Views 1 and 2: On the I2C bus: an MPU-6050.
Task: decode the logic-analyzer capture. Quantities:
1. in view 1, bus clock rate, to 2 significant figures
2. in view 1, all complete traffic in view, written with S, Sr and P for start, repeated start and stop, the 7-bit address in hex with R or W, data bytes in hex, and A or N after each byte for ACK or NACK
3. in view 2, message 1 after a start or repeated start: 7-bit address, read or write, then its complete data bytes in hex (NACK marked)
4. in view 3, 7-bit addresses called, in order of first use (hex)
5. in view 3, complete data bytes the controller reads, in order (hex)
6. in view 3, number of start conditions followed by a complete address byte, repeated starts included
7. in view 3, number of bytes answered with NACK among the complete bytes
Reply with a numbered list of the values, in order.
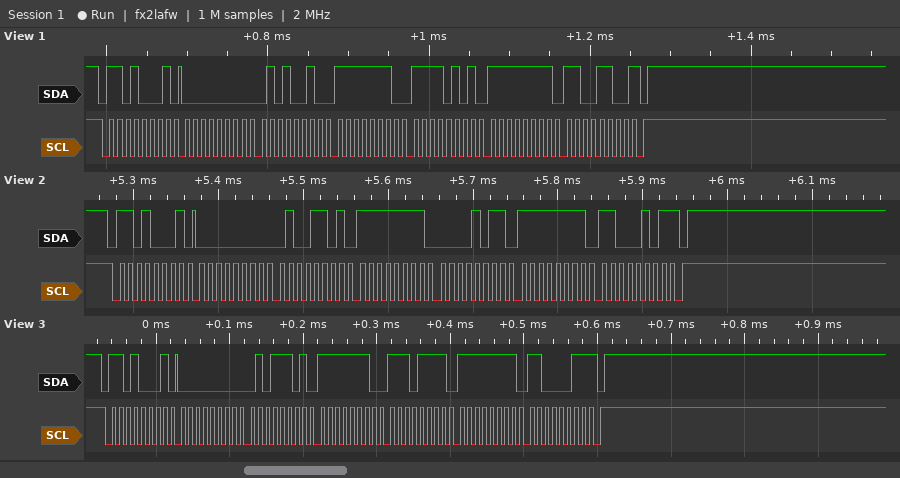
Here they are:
1. 100 kHz
2. S 68R A 00 A 52 A FE A F5 A FF A CC N P
3. 0x68 read: 00 4D FF 0B FF C5 NACK
4. 0x68
5. 00 5D FE EF FF C3
6. 1
7. 1
